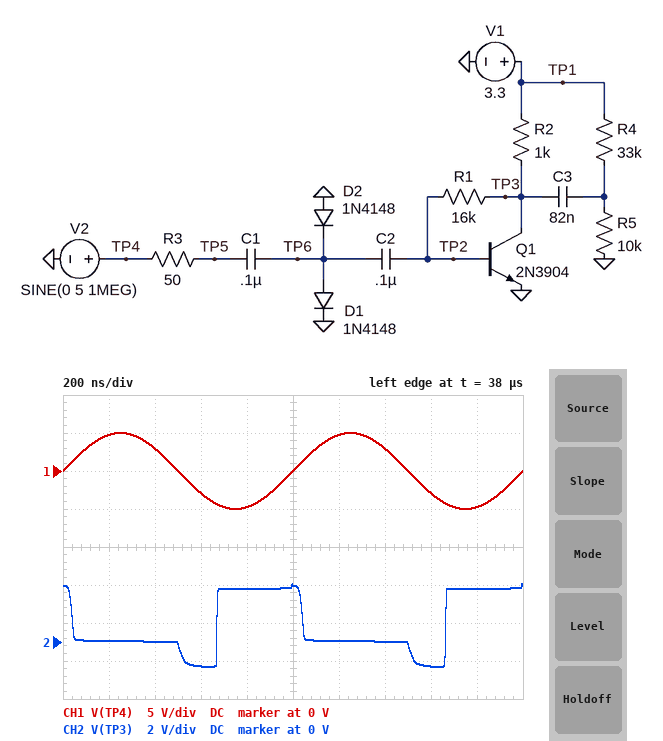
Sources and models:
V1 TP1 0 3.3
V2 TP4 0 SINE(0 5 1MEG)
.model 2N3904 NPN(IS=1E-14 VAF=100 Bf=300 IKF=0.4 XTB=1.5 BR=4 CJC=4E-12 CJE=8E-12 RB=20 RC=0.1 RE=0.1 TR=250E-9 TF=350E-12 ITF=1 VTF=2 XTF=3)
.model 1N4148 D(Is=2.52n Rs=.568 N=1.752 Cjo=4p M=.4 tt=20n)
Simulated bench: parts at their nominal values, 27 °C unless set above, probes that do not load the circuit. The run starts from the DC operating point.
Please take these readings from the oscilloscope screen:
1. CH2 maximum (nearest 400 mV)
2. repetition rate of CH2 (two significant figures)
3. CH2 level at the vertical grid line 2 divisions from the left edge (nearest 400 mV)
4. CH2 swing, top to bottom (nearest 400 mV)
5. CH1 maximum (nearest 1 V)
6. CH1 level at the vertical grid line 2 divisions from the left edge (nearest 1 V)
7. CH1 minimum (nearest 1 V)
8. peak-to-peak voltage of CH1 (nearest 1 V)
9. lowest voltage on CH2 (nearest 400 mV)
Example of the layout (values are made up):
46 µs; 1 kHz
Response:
3.2 V; 1.0 MHz; 0 V; 4.4 V; 5 V; 3 V; -5 V; 10 V; -1.2 V
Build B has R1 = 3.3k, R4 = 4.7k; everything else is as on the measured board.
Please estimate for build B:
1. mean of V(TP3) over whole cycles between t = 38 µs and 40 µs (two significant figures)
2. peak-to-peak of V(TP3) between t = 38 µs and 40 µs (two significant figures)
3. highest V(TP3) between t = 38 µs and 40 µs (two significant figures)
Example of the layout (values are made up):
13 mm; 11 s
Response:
590 mV; 3.6 V; 2.3 V
